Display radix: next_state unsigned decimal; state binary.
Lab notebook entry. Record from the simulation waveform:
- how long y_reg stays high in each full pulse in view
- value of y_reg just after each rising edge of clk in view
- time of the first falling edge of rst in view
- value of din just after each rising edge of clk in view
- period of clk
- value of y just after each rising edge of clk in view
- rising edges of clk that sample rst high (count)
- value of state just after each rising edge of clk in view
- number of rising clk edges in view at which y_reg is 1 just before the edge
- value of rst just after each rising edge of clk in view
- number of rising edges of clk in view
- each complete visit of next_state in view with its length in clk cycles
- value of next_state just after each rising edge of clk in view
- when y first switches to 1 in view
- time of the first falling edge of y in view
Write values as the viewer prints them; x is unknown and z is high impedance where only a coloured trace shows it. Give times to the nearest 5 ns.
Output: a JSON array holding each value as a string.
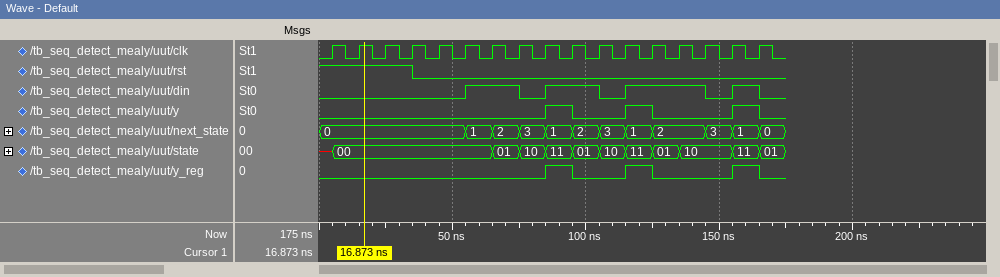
["10 ns, 10 ns, 10 ns", "0 0 0 0 0 0 0 0 1 0 0 1 0 0 0 1 0", "35 ns", "0 0 0 0 0 1 1 0 1 1 0 1 1 1 0 1 0", "10 ns", "0 0 0 0 0 0 0 0 1 0 0 1 0 0 0 1 0", "4", "00, 00, 00, 00, 00, 00, 01, 10, 11, 01, 10, 11, 01, 10, 10, 11, 01", "3", "1 1 1 0 0 0 0 0 0 0 0 0 0 0 0 0 0", "17", "1: 1, 2: 1, 3: 1, 1: 1, 2: 1, 3: 1, 1: 1, 2: 2, 3: 1, 1: 1", "0, 0, 0, 0, 0, 1, 2, 3, 1, 2, 3, 1, 2, 2, 3, 1, 0", "85 ns", "95 ns"]
